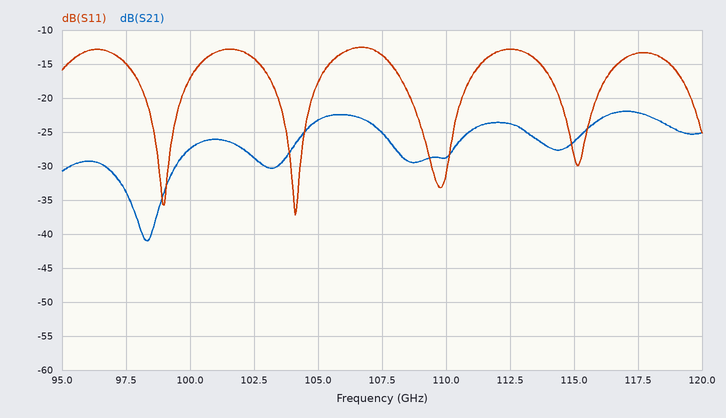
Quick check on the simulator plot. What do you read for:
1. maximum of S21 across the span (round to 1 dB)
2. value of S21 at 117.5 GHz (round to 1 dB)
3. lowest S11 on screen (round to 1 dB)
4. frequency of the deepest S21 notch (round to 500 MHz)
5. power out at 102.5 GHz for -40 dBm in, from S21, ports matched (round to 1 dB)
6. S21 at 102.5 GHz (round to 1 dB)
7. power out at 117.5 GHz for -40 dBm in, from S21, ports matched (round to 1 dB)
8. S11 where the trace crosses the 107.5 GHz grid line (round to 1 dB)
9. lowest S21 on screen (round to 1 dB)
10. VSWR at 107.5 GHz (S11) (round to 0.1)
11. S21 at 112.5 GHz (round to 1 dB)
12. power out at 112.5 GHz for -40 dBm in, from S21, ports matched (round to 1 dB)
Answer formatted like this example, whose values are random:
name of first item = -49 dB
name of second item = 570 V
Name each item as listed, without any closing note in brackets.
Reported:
maximum of S21 across the span = -22 dB
value of S21 at 117.5 GHz = -22 dB
lowest S11 on screen = -37 dB
frequency of the deepest S21 notch = 98.5 GHz
power out at 102.5 GHz for -40 dBm in, from S21, ports matched = -69 dBm
S21 at 102.5 GHz = -29 dB
power out at 117.5 GHz for -40 dBm in, from S21, ports matched = -62 dBm
S11 where the trace crosses the 107.5 GHz grid line = -14 dB
lowest S21 on screen = -41 dB
VSWR at 107.5 GHz (S11) = 1.5
S21 at 112.5 GHz = -24 dB
power out at 112.5 GHz for -40 dBm in, from S21, ports matched = -64 dBm
